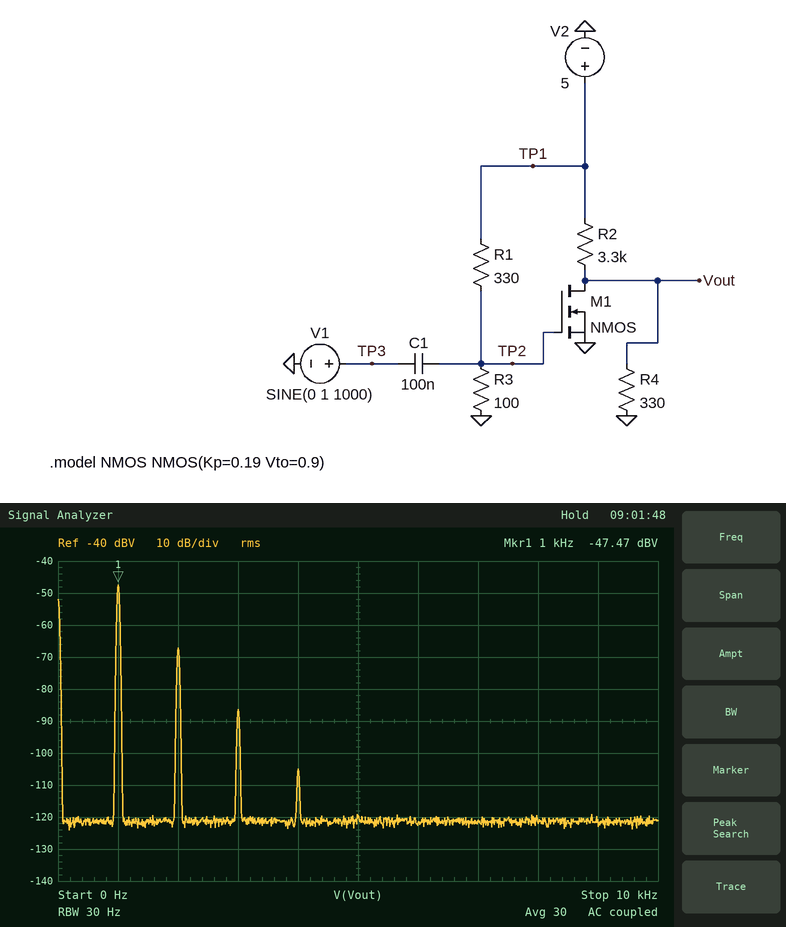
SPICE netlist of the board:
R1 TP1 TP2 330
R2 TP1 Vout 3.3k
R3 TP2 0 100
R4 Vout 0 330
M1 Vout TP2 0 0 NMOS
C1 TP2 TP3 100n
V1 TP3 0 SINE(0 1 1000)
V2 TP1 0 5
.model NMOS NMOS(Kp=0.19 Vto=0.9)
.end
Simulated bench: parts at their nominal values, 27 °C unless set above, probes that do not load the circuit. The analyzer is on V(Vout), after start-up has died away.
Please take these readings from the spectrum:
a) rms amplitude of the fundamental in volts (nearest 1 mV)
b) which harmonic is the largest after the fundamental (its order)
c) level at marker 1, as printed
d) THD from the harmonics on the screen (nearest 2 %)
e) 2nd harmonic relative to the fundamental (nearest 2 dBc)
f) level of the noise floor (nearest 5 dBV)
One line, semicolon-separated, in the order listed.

4 mV; 2; -47.47 dBV; 10 %; -20 dBc; -120 dBV
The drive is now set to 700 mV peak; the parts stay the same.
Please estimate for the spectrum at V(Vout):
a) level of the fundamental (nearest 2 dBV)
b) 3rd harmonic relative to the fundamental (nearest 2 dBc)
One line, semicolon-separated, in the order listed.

-50 dBV; -46 dBc
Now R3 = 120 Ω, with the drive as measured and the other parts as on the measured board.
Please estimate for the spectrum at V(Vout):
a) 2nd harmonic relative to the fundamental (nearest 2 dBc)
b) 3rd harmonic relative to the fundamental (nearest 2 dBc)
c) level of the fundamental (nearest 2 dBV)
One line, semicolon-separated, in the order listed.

-24 dBc; -48 dBc; -56 dBV
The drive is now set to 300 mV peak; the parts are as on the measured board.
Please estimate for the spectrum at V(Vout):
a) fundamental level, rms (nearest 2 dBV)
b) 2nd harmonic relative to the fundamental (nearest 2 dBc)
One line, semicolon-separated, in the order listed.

-58 dBV; -30 dBc
